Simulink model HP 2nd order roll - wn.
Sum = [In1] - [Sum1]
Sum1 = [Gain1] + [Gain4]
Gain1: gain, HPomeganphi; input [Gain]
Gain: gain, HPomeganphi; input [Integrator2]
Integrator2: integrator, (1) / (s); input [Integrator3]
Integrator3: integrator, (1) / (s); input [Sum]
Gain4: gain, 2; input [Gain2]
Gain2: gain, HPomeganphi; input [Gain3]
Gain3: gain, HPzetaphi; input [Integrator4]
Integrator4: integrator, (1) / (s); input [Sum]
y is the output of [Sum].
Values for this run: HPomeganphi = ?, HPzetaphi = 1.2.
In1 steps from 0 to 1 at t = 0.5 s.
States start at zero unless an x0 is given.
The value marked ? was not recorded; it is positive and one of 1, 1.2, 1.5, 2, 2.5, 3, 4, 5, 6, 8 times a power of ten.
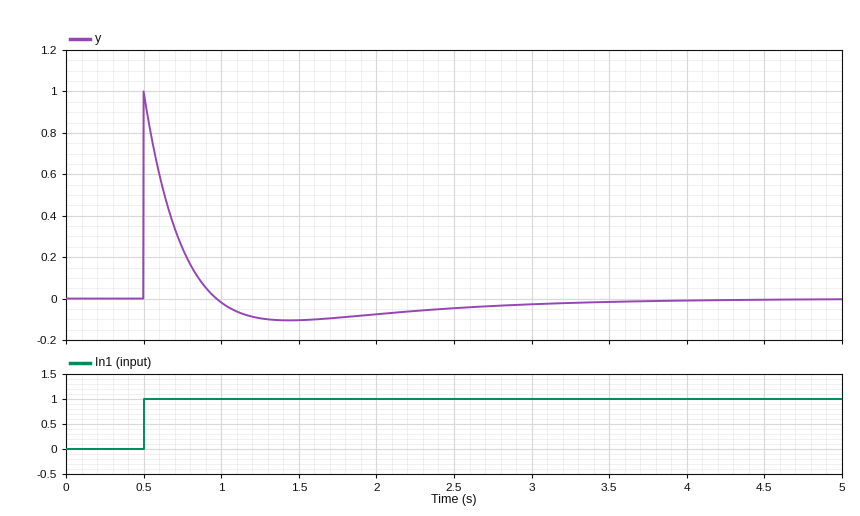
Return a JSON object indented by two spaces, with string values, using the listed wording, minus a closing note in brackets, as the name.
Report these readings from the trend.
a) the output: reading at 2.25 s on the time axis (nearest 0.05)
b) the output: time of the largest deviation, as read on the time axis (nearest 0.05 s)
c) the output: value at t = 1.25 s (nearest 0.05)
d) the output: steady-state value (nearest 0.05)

{
  "the output: reading at 2.25 s on the time axis": "-0.05",
  "the output: time of the largest deviation, as read on the time axis": "0.50 s",
  "the output: value at t = 1.25 s": "-0.10",
  "the output: steady-state value": "0.00"
}
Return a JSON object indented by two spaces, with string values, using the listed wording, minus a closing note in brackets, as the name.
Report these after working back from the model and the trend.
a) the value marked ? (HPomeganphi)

{
  "the value marked ?": "2"
}
